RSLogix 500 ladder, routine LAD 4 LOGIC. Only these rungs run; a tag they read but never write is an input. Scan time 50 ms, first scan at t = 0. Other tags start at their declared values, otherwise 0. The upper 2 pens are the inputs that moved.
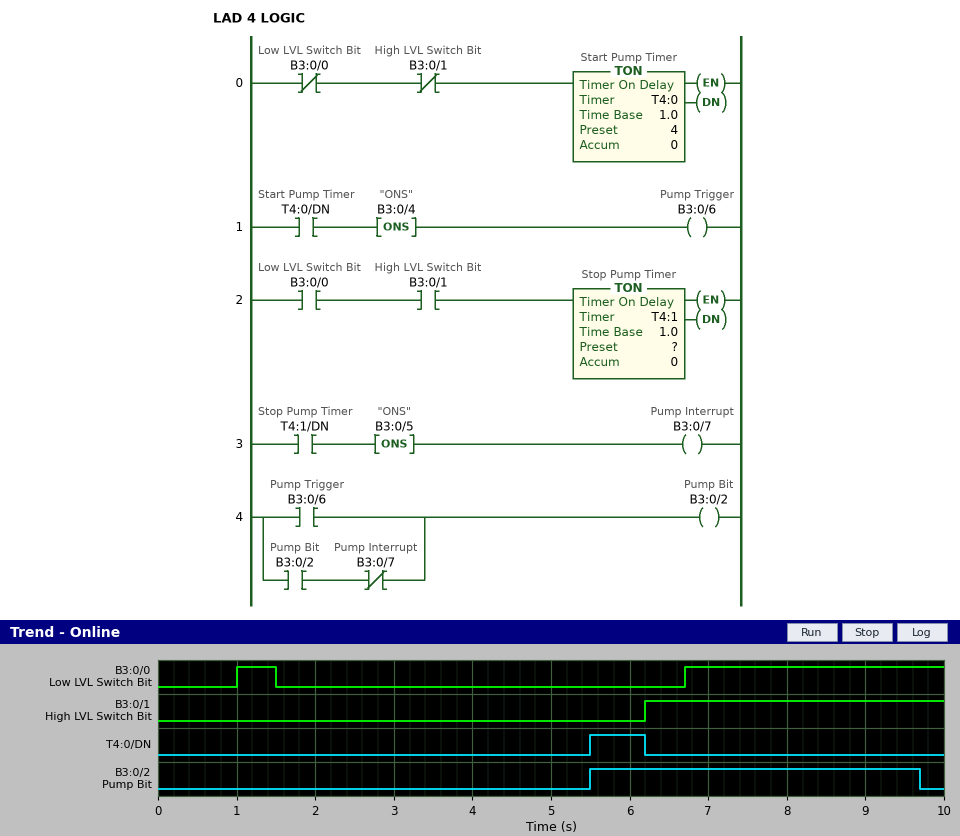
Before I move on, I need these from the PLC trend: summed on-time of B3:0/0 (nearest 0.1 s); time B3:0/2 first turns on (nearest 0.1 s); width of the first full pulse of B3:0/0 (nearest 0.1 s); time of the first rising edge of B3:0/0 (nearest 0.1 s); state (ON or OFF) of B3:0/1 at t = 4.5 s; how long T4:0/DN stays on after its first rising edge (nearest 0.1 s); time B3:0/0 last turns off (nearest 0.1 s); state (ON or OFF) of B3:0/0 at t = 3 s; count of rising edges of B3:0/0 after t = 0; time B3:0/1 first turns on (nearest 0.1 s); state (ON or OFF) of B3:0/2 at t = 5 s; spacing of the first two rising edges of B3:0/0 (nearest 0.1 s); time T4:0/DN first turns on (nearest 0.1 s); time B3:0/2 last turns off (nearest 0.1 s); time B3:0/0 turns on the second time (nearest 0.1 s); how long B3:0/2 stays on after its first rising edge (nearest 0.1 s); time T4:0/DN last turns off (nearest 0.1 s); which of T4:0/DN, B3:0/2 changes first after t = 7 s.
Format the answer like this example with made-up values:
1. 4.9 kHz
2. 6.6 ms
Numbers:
1. 3.8 s
2. 5.5 s
3. 0.5 s
4. 1.0 s
5. OFF
6. 0.7 s
7. 1.5 s
8. OFF
9. 2
10. 6.2 s
11. OFF
12. 5.7 s
13. 5.5 s
14. 9.7 s
15. 6.7 s
16. 4.2 s
17. 6.2 s
18. B3:0/2
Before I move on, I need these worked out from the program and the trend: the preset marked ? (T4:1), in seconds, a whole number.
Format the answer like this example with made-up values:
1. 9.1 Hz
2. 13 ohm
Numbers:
1. 3 s
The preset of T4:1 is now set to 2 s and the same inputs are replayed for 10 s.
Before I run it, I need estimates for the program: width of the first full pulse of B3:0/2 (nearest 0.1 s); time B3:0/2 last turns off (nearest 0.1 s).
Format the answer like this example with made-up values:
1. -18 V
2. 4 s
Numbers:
1. 3.2 s
2. 8.7 s
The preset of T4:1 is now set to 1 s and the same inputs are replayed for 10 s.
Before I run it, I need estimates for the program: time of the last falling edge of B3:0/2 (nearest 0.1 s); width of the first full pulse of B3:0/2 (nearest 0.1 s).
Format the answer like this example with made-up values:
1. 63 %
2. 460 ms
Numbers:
1. 7.7 s
2. 2.2 s
